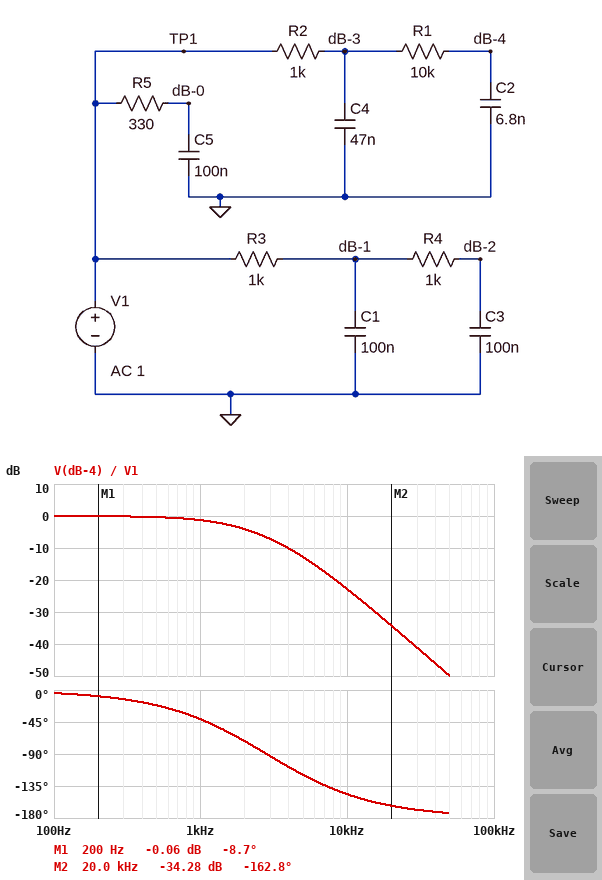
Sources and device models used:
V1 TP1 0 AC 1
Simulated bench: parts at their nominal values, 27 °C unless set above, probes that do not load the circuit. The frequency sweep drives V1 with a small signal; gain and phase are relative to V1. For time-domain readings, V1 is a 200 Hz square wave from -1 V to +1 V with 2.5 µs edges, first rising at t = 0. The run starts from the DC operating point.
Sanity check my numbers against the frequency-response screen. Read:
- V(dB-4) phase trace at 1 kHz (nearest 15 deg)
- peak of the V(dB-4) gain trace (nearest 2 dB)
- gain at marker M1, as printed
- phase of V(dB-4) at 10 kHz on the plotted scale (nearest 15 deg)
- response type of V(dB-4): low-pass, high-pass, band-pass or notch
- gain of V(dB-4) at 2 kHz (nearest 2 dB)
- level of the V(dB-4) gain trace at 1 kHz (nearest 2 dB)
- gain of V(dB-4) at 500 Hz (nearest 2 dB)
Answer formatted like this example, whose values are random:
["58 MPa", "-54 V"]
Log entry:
["-45 deg", "0 dB", "-0.06 dB", "-150 deg", "low-pass", "-4 dB", "-2 dB", "0 dB"]
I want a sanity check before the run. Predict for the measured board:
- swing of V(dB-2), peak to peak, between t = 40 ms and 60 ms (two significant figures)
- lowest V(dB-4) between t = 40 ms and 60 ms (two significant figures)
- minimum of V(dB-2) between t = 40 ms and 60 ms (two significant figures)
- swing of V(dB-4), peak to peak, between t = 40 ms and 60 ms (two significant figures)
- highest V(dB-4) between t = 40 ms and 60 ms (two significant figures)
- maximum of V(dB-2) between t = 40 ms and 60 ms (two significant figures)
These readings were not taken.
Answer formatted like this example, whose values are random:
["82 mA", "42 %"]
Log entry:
["2.0 V", "-1.0 V", "-1.0 V", "2.0 V", "1.0 V", "1.0 V"]
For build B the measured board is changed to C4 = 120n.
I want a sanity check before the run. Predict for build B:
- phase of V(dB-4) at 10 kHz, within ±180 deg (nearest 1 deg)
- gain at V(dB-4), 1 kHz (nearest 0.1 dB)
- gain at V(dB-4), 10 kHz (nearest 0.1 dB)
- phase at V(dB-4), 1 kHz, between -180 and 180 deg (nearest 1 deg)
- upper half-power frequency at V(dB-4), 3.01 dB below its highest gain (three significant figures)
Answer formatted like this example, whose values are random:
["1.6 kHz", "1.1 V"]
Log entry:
["-159 deg", "-2.9 dB", "-30.5 dB", "-61 deg", "1.02 kHz"]
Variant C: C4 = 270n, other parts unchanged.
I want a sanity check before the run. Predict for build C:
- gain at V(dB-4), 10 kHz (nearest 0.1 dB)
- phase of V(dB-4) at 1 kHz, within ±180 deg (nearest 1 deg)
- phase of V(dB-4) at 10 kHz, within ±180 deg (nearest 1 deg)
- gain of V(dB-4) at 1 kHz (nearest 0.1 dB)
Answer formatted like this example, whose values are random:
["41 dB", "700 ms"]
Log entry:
["-37.5 dB", "-83 deg", "-163 deg", "-6.8 dB"]
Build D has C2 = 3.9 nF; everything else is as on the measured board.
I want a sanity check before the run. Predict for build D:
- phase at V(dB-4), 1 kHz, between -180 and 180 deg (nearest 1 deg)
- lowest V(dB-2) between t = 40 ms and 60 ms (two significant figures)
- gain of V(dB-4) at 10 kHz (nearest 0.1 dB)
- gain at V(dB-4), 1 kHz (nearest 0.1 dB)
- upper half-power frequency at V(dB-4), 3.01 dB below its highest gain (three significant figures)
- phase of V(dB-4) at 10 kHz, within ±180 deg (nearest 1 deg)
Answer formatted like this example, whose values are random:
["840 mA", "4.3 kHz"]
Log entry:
["-31 deg", "-1.0 V", "-18.5 dB", "-0.7 dB", "2.23 kHz", "-138 deg"]
